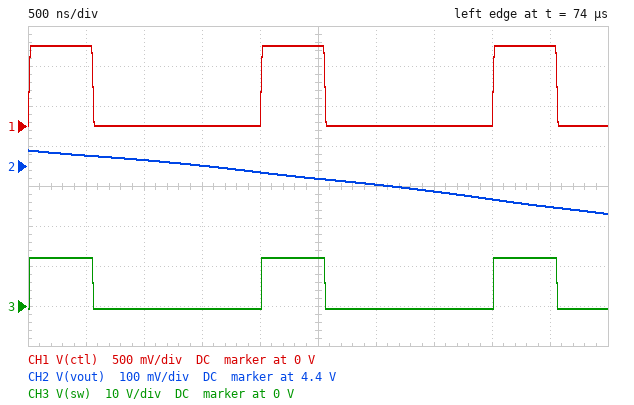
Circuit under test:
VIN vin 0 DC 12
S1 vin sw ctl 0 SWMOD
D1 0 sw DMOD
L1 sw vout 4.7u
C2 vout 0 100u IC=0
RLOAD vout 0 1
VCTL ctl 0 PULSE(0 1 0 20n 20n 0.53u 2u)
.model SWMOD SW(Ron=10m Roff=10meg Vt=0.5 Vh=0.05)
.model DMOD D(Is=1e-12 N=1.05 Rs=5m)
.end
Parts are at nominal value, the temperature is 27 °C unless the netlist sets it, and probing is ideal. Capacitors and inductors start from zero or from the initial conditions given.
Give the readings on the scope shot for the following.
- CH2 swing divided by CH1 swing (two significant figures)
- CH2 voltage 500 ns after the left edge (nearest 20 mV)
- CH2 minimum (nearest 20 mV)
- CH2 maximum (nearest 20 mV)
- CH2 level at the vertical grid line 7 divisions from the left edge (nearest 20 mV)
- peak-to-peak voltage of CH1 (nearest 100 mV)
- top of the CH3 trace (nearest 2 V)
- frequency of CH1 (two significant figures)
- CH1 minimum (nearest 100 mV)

0.16
4.42 V
4.28 V
4.44 V
4.34 V
1.0 V
12 V
500 kHz
0 V
